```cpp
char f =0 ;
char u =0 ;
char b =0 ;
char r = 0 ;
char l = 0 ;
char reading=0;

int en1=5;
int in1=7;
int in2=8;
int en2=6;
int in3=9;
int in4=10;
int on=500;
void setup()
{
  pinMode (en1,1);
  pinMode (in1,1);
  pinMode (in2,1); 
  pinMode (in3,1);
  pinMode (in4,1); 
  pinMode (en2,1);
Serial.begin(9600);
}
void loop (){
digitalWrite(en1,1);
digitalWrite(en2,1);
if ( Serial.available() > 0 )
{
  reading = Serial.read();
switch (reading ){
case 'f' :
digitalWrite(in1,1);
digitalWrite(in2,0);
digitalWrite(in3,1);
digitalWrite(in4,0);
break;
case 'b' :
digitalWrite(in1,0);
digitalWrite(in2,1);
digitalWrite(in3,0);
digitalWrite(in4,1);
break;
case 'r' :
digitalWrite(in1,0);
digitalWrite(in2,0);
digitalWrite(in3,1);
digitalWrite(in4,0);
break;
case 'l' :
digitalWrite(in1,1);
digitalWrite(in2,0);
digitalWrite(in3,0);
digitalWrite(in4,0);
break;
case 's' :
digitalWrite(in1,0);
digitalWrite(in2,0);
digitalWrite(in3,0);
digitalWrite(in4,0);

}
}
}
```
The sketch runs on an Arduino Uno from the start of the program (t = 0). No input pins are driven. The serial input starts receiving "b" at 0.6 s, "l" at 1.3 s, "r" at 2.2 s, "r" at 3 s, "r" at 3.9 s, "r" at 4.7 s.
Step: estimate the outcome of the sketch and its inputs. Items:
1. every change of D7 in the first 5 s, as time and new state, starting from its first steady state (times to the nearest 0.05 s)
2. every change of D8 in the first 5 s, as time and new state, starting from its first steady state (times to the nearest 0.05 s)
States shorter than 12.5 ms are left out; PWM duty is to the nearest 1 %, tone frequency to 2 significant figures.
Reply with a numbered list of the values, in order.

1. 0 s low; 1.3 s high; 2.2 s low
2. 0 s low; 0.6 s high; 1.3 s low
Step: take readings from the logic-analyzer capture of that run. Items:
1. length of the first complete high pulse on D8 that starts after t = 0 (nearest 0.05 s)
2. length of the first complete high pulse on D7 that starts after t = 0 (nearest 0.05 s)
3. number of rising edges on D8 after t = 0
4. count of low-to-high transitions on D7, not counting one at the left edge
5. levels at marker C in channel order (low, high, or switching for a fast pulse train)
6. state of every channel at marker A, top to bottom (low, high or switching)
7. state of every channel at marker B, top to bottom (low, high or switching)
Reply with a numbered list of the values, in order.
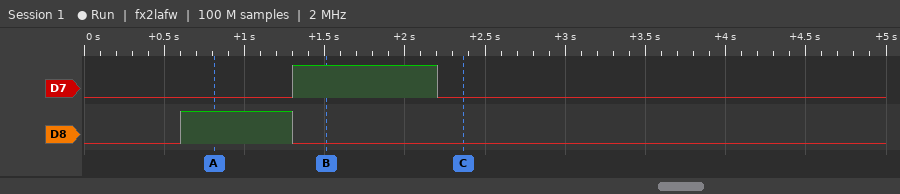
1. 0.70 s
2. 0.90 s
3. 1
4. 1
5. D7 low, D8 low
6. D7 low, D8 high
7. D7 high, D8 low
